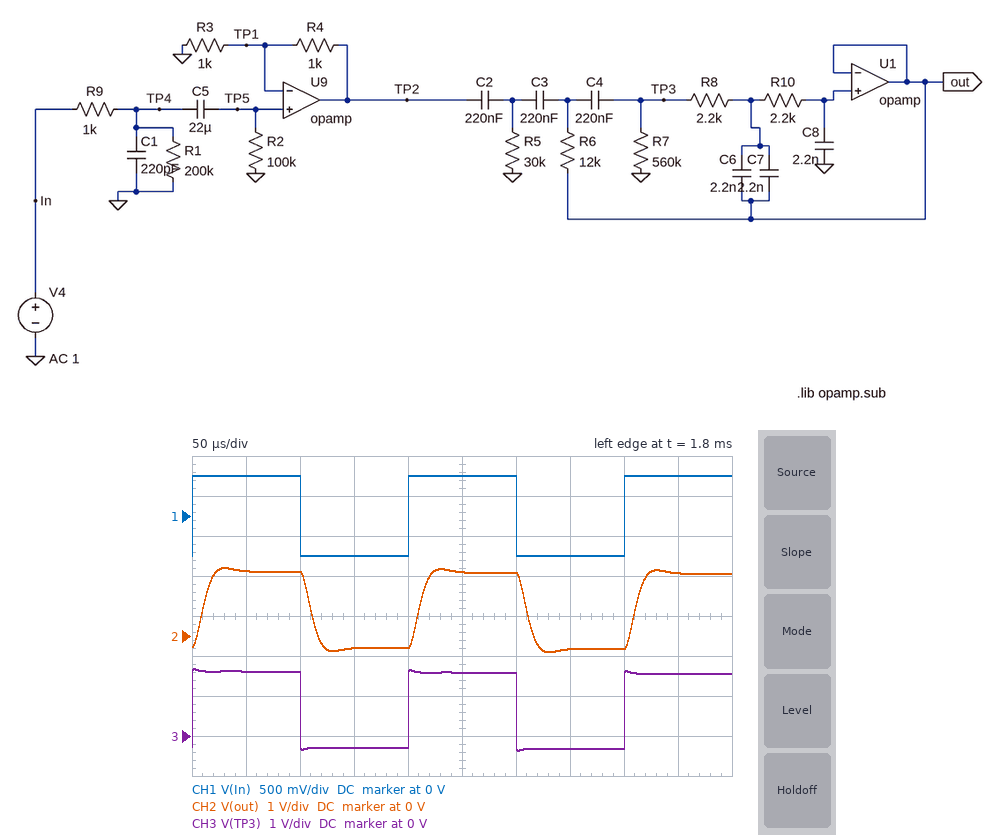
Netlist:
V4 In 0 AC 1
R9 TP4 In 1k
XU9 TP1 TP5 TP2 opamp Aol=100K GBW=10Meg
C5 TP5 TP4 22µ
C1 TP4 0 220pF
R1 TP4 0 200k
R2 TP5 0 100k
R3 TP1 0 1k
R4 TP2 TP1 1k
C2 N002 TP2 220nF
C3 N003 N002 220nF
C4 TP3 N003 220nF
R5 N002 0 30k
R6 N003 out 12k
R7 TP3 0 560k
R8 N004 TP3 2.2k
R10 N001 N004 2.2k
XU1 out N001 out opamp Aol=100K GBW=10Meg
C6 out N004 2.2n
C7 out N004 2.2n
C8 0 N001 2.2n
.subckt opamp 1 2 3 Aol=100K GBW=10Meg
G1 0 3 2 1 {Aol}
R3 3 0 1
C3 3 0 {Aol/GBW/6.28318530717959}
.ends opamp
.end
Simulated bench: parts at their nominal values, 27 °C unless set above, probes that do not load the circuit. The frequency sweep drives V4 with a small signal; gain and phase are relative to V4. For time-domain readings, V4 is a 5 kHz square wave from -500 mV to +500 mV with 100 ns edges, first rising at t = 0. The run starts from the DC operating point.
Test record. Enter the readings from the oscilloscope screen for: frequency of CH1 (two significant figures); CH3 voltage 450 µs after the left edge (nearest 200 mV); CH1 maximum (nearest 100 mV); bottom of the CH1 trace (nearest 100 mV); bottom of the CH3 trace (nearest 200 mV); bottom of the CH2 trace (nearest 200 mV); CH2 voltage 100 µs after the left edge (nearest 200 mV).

5.0 kHz
1.6 V
500 mV
-500 mV
-400 mV
-400 mV
1.6 V
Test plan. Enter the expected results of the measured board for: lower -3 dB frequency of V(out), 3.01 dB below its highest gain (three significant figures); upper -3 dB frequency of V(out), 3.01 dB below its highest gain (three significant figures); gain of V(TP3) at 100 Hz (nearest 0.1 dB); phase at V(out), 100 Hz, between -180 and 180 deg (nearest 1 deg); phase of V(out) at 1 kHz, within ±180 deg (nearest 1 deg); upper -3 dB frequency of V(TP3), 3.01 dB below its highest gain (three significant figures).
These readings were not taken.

13.3 Hz
23.3 kHz
5.4 dB
16 deg
-2 deg
731 kHz
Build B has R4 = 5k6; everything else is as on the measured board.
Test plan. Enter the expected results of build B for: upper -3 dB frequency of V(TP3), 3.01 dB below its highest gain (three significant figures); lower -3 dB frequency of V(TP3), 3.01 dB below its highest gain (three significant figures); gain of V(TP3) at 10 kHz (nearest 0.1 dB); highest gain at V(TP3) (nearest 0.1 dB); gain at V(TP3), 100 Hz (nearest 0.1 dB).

630 kHz
15.0 Hz
15.9 dB
16.2 dB
15.8 dB
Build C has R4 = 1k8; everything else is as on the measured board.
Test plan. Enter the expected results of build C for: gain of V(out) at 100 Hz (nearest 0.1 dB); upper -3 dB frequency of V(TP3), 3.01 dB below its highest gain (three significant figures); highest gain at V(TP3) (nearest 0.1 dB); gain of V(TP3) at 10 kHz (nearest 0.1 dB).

8.3 dB
718 kHz
8.7 dB
8.5 dB
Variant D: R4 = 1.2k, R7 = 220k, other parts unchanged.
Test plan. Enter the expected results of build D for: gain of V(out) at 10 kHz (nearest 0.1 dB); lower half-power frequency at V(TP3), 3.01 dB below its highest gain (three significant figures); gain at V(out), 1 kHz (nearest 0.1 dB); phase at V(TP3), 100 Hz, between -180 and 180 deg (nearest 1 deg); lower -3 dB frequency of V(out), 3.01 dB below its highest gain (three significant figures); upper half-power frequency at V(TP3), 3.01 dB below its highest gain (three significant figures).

6.2 dB
17.4 Hz
6.4 dB
20 deg
17.0 Hz
728 kHz
